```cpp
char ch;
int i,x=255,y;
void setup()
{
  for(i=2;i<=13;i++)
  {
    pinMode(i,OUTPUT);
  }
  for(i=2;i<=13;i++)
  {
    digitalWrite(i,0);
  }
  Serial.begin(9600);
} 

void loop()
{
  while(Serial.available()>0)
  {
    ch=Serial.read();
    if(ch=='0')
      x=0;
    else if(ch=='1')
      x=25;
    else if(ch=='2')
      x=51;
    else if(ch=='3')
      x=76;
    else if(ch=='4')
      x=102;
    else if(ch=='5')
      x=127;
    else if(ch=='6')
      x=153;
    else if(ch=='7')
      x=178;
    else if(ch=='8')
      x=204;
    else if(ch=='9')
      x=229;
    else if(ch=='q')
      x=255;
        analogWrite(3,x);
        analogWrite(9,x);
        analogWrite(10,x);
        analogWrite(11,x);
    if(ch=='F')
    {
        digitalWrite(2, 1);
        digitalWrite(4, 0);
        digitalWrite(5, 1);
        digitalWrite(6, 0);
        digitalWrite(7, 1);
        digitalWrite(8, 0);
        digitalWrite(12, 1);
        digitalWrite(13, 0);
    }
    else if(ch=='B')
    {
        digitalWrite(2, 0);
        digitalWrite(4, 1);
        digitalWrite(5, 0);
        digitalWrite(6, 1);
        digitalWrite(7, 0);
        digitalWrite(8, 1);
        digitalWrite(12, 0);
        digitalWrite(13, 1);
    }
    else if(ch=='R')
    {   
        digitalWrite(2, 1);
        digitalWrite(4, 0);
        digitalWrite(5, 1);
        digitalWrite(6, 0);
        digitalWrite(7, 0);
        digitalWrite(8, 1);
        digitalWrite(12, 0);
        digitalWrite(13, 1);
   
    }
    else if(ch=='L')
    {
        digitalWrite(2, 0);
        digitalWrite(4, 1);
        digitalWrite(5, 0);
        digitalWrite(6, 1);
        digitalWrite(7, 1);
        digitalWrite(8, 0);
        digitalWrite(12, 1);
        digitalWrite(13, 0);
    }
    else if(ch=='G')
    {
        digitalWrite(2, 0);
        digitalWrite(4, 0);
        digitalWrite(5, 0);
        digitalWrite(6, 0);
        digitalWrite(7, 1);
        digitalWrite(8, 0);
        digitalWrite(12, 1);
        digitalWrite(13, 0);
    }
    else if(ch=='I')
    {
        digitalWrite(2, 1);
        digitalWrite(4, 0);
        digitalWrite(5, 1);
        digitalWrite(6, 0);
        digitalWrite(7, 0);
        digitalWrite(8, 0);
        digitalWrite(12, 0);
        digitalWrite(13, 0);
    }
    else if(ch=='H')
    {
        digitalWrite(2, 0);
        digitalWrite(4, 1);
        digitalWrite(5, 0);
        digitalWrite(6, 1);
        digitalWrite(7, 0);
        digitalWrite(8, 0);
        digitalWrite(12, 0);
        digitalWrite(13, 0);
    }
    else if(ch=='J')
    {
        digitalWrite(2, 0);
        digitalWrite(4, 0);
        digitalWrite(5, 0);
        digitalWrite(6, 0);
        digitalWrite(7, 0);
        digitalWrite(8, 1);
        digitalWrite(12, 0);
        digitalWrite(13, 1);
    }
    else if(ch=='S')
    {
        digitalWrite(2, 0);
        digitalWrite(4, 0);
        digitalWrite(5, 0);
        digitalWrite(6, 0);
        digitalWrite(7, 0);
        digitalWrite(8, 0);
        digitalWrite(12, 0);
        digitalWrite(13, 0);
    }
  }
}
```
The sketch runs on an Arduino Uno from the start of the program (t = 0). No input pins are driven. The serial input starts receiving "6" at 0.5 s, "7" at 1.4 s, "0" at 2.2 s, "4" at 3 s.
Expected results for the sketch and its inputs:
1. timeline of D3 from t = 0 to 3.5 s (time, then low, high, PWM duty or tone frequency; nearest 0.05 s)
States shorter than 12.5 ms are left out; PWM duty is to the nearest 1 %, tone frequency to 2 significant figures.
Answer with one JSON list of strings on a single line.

["0 s low; 0.5 s PWM 60 %; 1.4 s PWM 70 %; 2.2 s low; 3 s PWM 40 %"]
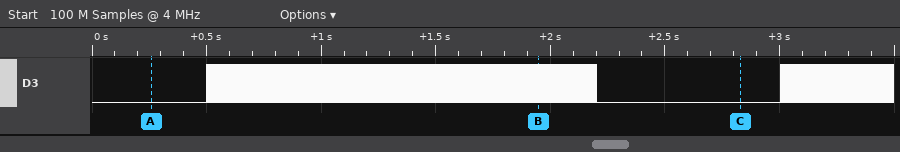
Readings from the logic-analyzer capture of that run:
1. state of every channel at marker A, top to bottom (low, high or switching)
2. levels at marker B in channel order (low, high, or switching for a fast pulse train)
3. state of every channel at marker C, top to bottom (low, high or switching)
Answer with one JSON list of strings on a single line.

["D3 low", "D3 switching", "D3 low"]
